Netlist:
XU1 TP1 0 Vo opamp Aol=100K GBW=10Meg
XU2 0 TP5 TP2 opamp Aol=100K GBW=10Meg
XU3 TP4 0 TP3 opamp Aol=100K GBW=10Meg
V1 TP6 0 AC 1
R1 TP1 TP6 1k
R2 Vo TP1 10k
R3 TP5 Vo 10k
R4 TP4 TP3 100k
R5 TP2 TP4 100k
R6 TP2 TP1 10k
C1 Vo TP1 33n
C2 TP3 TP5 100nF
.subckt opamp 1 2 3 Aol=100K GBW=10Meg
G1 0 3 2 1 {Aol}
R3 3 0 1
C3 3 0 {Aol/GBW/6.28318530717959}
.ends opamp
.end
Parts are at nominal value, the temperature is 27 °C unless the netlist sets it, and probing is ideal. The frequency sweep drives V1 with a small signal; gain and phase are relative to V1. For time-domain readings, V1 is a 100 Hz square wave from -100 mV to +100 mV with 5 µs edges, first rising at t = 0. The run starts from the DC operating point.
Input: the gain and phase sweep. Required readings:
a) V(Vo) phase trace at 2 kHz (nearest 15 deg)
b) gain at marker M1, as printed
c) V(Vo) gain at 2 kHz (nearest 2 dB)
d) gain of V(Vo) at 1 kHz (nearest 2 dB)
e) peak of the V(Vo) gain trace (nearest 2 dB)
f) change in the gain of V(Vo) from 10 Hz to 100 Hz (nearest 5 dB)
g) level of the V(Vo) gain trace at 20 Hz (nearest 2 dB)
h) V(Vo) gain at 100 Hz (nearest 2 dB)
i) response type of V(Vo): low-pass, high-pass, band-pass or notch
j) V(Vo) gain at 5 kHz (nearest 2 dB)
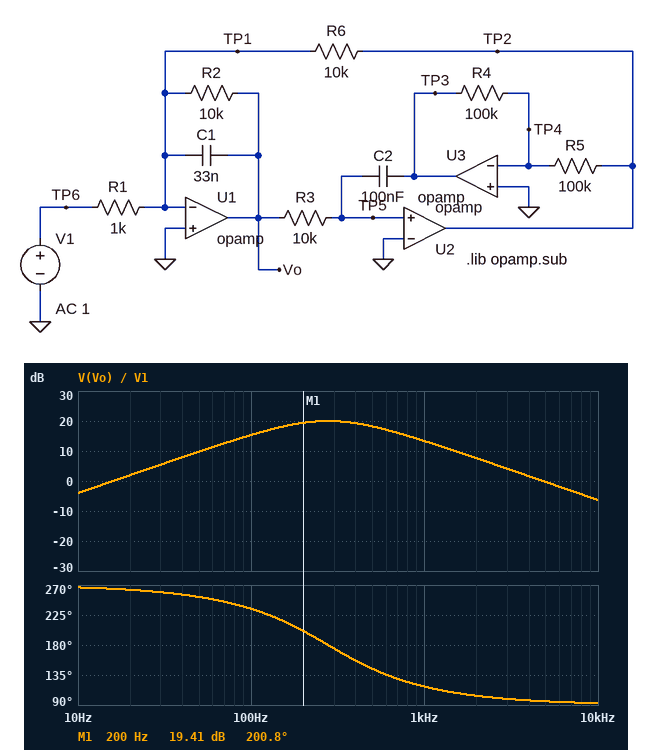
105 deg
19.41 dB
8 dB
14 dB
20 dB
20 dB
2 dB
16 dB
band-pass
0 dB
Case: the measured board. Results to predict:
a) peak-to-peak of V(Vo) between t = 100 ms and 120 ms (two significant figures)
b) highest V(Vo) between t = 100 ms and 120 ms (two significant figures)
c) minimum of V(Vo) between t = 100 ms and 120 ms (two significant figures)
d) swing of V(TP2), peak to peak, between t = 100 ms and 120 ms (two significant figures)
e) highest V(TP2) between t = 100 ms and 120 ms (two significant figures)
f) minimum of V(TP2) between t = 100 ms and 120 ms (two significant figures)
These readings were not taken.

2.8 V
1.4 V
-1.4 V
2.0 V
1.0 V
-1.0 V
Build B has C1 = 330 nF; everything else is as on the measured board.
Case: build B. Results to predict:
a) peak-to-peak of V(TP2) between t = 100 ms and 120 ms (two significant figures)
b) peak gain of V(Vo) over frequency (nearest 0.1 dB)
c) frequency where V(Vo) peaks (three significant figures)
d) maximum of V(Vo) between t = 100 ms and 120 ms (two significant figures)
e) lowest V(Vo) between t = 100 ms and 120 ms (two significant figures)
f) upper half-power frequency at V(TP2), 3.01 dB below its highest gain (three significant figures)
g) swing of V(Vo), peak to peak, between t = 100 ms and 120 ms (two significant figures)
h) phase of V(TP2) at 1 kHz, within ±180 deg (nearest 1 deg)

3.7 V
20.0 dB
87.6 Hz
1.1 V
-1.1 V
103 Hz
2.2 V
3 deg
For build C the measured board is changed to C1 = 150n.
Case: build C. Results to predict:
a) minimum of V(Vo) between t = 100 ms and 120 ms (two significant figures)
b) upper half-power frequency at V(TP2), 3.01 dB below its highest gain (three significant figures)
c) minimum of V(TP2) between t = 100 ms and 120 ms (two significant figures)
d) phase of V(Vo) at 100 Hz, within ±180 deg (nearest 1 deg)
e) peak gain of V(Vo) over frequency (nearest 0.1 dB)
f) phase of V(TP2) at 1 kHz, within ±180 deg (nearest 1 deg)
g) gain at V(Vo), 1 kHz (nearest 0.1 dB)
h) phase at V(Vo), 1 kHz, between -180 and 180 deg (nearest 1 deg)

-1.2 V
154 Hz
-1.6 V
-147 deg
20.0 dB
6 deg
0.6 dB
96 deg
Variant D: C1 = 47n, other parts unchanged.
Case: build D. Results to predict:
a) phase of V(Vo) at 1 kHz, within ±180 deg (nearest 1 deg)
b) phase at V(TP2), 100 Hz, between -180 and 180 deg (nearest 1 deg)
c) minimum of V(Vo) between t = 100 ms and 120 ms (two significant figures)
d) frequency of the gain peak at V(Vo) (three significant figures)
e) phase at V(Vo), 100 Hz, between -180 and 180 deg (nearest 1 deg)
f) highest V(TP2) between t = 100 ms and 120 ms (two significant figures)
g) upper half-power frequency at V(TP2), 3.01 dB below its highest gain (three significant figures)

110 deg
142 deg
-1.3 V
232 Hz
-128 deg
1.1 V
225 Hz
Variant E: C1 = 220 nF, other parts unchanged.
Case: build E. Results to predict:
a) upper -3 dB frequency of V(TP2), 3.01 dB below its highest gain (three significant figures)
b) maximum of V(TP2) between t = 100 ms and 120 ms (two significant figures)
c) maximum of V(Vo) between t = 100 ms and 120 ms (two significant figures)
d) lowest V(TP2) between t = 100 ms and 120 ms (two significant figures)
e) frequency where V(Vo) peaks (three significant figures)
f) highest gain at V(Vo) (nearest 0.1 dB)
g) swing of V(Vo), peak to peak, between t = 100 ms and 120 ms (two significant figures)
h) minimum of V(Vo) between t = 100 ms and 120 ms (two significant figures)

127 Hz
2.0 V
1.3 V
-2.0 V
107 Hz
20.0 dB
2.6 V
-1.3 V
